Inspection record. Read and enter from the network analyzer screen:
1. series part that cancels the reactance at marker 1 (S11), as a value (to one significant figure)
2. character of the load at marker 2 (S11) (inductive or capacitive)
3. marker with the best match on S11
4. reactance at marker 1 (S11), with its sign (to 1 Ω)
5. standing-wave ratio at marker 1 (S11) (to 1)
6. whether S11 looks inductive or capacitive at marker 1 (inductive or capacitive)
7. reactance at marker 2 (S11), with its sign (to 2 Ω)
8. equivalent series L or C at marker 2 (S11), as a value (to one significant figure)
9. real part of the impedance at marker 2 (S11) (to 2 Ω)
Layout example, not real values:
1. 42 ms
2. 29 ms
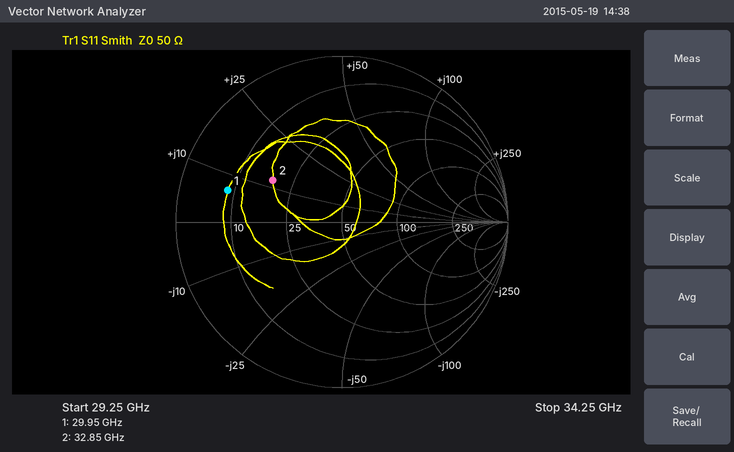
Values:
1. 800 fF
2. inductive
3. marker 2
4. +7 Ω
5. 6
6. inductive
7. +12 Ω
8. 60 pH
9. 18 Ω
